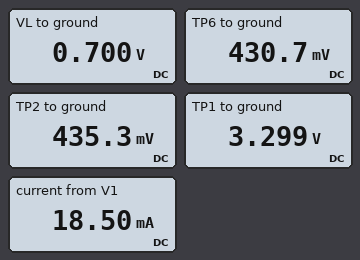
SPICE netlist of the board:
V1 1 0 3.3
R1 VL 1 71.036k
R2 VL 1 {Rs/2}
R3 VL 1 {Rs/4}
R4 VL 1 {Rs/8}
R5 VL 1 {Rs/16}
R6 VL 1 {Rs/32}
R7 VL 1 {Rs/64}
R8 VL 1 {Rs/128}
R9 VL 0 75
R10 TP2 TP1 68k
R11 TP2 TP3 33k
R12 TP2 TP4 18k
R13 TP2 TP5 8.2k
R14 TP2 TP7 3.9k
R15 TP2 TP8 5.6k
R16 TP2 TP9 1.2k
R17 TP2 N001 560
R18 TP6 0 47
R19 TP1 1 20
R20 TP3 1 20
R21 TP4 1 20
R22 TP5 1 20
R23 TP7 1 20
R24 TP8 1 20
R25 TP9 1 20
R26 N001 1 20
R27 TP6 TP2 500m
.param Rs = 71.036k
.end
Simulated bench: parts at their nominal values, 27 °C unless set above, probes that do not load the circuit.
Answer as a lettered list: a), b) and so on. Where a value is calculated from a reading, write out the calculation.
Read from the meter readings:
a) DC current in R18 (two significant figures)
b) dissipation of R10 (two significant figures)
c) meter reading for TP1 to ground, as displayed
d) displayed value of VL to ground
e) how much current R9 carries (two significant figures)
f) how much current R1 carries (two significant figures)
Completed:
a) (430.7 mV) / 47 Ω = 9.2 mA
b) (3.299 V - 435.3 mV)^2 / 68 kΩ = 120 µW
c) 3.299 V
d) 0.700 V
e) (700 mV) / 75 Ω = 9.3 mA
f) (3.3 V - 700 mV) / 71.04 kΩ = 37 µA
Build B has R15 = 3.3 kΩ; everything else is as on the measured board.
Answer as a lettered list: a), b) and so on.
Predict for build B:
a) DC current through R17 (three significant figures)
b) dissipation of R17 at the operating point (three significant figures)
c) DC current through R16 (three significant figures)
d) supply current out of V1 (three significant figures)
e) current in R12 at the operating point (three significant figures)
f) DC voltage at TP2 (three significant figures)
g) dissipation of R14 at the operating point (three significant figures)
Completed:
a) 4.91 mA
b) 13.5 mW
c) 2.34 mA
d) 18.8 mA
e) 158 µA
f) 450 mV
g) 2.06 mW
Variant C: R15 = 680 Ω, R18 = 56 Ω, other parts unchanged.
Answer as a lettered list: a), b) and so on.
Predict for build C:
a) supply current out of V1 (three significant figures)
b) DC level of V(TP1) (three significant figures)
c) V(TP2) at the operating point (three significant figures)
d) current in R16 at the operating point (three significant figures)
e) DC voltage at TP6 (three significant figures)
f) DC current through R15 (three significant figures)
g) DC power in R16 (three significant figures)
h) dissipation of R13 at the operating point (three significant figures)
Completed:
a) 21.1 mA
b) 3.30 V
c) 663 mV
d) 2.16 mA
e) 657 mV
f) 3.77 mA
g) 5.61 mW
h) 844 µW
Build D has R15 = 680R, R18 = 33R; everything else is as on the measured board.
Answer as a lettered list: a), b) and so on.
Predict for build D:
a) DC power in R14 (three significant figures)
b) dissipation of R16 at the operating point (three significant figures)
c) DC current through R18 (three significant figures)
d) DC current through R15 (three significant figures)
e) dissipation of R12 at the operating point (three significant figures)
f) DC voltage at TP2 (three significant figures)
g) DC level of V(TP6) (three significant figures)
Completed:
a) 2.09 mW
b) 6.65 mW
c) 12.8 mA
d) 4.10 mA
e) 457 µW
f) 428 mV
g) 422 mV
